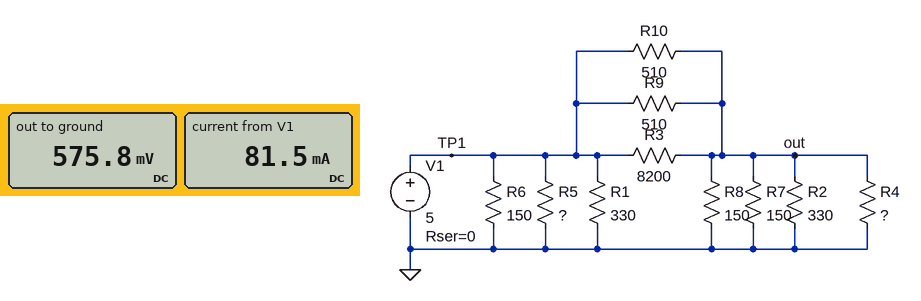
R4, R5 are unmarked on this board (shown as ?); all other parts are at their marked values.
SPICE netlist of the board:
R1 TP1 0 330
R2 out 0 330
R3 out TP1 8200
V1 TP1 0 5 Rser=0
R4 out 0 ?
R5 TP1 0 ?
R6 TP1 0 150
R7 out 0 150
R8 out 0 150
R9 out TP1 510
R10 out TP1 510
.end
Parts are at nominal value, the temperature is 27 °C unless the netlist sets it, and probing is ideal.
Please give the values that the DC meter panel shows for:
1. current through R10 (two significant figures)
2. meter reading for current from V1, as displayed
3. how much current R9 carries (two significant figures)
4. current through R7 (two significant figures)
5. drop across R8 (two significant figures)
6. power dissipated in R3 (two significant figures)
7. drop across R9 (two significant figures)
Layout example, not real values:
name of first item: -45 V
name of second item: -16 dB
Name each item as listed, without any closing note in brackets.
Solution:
current through R10: 8.7 mA
meter reading for current from V1, as displayed: 81.5 mA
how much current R9 carries: 8.7 mA
current through R7: 3.8 mA
drop across R8: 580 mV
power dissipated in R3: 2.4 mW
drop across R9: 4.4 V
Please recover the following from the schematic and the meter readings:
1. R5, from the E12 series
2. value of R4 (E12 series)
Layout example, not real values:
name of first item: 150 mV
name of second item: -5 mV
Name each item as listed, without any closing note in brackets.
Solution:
R5, from the E12 series: 330 Ω
value of R4: 68 Ω
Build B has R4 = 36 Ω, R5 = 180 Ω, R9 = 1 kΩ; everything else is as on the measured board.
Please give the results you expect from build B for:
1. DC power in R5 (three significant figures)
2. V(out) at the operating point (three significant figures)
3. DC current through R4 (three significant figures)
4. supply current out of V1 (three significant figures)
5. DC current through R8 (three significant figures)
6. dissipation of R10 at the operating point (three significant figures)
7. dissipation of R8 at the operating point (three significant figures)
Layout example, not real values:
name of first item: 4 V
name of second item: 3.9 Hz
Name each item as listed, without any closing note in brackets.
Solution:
DC power in R5: 139 mW
V(out) at the operating point: 326 mV
DC current through R4: 9.07 mA
supply current out of V1: 90.7 mA
DC current through R8: 2.18 mA
dissipation of R10 at the operating point: 42.8 mW
dissipation of R8 at the operating point: 710 µW
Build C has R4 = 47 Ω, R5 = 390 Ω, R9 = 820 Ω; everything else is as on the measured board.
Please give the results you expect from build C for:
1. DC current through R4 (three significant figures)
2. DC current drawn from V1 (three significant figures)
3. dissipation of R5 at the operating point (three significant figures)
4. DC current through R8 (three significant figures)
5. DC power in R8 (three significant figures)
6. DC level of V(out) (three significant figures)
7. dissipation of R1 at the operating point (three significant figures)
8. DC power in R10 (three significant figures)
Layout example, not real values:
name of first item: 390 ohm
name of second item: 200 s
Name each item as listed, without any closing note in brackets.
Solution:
DC current through R4: 8.58 mA
DC current drawn from V1: 76.5 mA
dissipation of R5 at the operating point: 64.1 mW
DC current through R8: 2.69 mA
DC power in R8: 1.08 mW
DC level of V(out): 403 mV
dissipation of R1 at the operating point: 75.8 mW
DC power in R10: 41.4 mW
